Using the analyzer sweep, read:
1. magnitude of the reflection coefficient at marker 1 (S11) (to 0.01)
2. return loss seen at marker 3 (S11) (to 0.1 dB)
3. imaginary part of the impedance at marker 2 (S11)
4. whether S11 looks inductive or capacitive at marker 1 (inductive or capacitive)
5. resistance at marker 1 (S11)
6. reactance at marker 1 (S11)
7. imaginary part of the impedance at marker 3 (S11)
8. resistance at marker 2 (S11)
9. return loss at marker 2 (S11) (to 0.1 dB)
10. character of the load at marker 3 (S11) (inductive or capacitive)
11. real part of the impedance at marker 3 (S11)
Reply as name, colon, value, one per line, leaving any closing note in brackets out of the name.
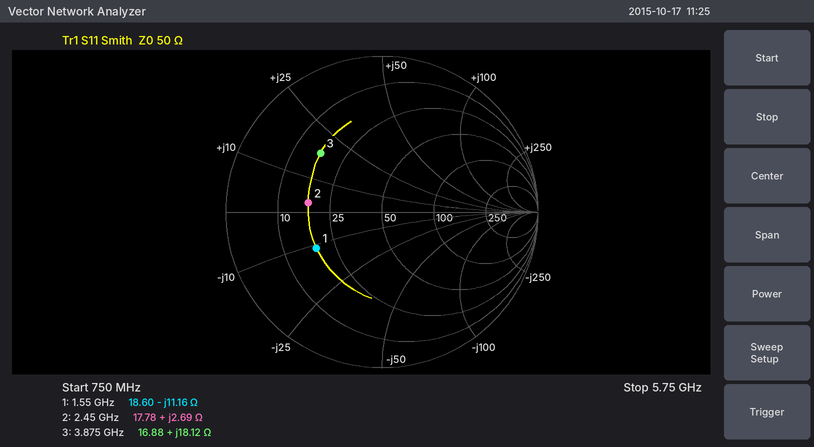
magnitude of the reflection coefficient at marker 1 (S11): 0.48
return loss seen at marker 3 (S11): 5.3 dB
imaginary part of the impedance at marker 2: +2.69 Ω
whether S11 looks inductive or capacitive at marker 1: capacitive
resistance at marker 1: 18.60 Ω
reactance at marker 1: -11.16 Ω
imaginary part of the impedance at marker 3: +18.12 Ω
resistance at marker 2: 17.78 Ω
return loss at marker 2 (S11): 6.4 dB
character of the load at marker 3 (S11): inductive
real part of the impedance at marker 3: 16.88 Ω
